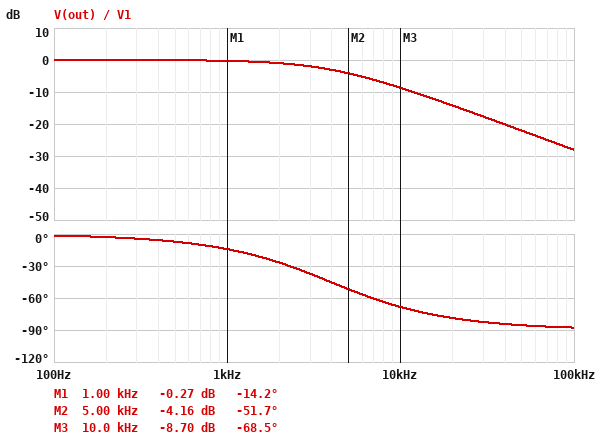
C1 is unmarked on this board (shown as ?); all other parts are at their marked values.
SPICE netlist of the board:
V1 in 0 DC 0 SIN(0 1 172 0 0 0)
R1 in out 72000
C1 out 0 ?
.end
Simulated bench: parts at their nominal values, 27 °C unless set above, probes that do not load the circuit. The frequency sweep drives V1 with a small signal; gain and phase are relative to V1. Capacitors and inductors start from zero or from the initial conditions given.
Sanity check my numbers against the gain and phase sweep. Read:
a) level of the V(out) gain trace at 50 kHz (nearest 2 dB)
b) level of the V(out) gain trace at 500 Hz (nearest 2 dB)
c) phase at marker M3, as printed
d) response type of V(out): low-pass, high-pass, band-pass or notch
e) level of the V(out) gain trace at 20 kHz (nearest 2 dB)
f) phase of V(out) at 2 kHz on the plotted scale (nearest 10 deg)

-22 dB
0 dB
-68.5 deg
low-pass
-14 dB
-30 deg
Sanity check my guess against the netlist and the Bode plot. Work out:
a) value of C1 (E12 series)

560 pF
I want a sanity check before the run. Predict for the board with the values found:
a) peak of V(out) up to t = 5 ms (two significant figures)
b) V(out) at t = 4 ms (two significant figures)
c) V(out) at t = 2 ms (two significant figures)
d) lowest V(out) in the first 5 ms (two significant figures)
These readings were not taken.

1.0 V
-910 mV
850 mV
-1.0 V
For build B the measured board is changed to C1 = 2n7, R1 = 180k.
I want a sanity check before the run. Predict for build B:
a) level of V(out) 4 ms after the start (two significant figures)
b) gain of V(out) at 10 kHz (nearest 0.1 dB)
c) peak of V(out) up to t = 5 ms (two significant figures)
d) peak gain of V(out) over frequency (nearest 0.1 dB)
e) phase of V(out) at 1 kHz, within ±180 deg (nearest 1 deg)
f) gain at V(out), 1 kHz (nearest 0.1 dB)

-570 mV
-29.7 dB
890 mV
0 dB
-72 deg
-10.1 dB
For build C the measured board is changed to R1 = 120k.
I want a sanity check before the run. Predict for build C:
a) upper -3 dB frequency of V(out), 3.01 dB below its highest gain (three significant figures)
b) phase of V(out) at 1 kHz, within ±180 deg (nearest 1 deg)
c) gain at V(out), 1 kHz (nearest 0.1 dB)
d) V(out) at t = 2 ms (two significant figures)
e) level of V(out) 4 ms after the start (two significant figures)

2.37 kHz
-23 deg
-0.7 dB
870 mV
-890 mV
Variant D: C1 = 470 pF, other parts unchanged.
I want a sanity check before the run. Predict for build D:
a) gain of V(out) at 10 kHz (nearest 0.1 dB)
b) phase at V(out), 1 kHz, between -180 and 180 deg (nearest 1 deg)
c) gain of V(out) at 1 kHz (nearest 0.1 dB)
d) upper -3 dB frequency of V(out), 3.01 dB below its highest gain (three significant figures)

-7.4 dB
-12 deg
-0.2 dB
4.70 kHz
